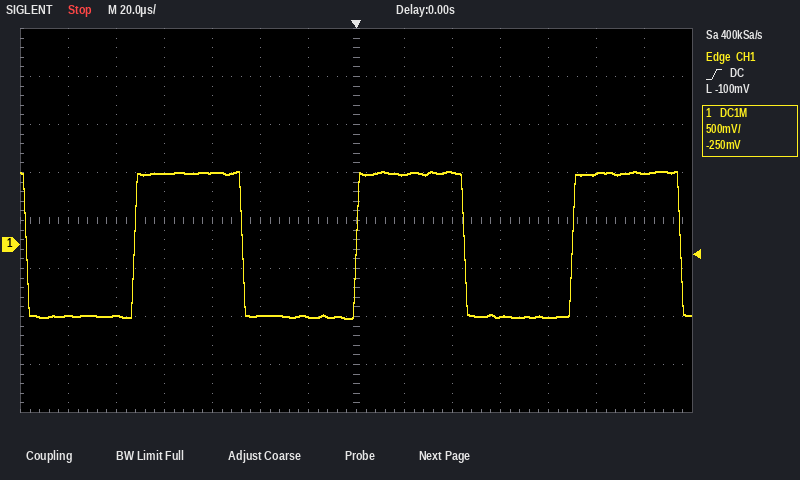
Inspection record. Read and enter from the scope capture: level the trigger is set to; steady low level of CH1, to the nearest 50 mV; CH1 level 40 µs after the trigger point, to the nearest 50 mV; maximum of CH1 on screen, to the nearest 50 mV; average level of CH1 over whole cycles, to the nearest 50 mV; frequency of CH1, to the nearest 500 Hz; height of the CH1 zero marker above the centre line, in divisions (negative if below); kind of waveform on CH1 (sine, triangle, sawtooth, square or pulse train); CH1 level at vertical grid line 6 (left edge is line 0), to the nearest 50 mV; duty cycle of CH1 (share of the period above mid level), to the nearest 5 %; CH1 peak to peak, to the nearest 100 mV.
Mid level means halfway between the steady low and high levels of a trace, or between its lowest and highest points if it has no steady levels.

-100 mV
-750 mV
750 mV
750 mV
0 mV
11.0 kHz
-0.5 div
square
-750 mV
50 %
1.50 V
